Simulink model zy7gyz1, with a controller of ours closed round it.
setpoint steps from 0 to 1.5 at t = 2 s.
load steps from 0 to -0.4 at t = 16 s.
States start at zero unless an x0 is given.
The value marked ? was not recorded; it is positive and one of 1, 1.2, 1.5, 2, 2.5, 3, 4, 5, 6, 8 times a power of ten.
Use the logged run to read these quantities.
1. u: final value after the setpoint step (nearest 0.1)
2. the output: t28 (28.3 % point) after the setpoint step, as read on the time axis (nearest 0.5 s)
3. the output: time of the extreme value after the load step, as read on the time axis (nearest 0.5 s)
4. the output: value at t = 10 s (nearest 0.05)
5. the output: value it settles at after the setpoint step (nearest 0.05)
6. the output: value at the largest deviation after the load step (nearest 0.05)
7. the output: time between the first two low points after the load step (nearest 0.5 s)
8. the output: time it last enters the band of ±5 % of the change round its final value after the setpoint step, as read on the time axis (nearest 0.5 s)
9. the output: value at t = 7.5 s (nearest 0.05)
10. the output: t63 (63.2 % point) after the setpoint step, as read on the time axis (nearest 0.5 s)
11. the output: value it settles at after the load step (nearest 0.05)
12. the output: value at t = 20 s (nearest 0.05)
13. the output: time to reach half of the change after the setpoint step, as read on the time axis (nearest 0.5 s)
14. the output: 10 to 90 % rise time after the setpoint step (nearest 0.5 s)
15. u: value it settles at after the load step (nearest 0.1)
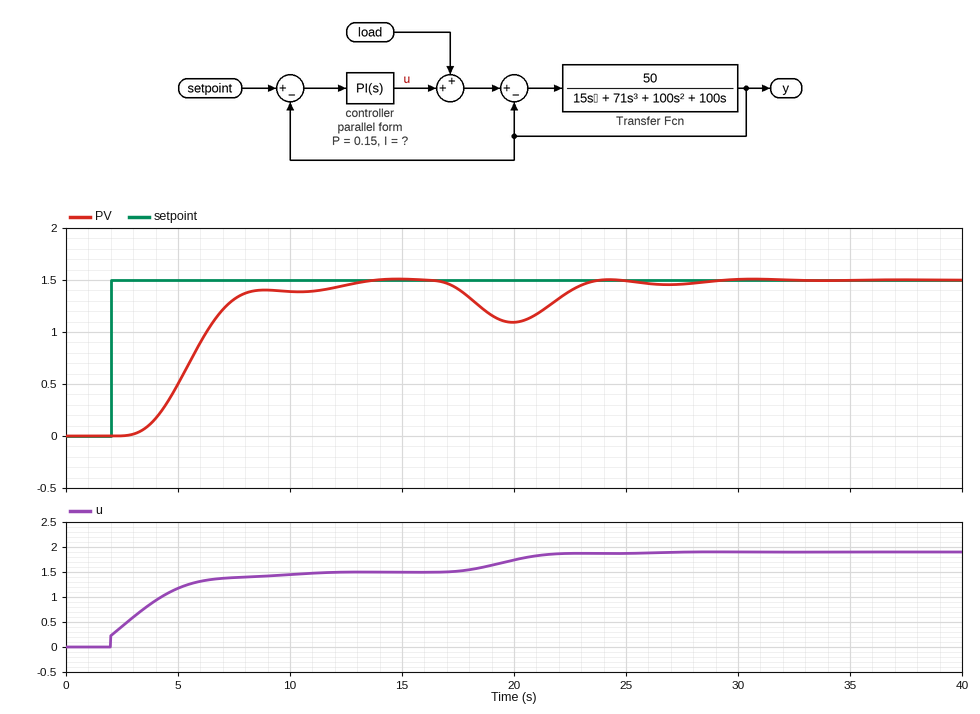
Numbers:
1.5
5.0 s
20.0 s
1.40
1.50
1.10
7.0 s
12.0 s
1.30
6.0 s
1.50
1.10
5.5 s
4.0 s
1.9
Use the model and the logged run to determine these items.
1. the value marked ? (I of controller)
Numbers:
0.25
